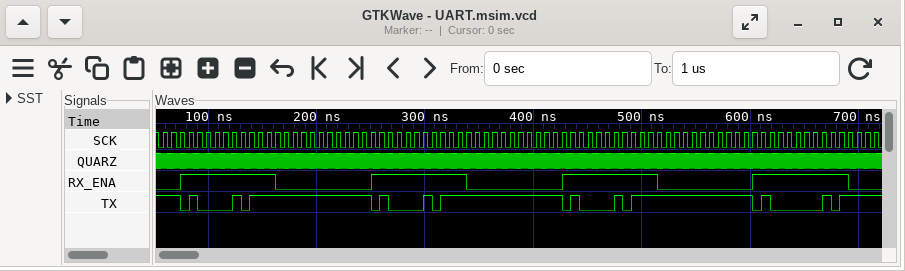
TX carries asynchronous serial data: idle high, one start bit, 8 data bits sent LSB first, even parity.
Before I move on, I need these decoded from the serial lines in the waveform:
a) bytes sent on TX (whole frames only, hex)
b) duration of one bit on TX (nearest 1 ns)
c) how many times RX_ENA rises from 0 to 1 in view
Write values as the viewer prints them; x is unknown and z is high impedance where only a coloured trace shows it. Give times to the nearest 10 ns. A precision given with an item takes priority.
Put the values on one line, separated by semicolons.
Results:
A1, A1, A1, 81; 8 ns; 4
